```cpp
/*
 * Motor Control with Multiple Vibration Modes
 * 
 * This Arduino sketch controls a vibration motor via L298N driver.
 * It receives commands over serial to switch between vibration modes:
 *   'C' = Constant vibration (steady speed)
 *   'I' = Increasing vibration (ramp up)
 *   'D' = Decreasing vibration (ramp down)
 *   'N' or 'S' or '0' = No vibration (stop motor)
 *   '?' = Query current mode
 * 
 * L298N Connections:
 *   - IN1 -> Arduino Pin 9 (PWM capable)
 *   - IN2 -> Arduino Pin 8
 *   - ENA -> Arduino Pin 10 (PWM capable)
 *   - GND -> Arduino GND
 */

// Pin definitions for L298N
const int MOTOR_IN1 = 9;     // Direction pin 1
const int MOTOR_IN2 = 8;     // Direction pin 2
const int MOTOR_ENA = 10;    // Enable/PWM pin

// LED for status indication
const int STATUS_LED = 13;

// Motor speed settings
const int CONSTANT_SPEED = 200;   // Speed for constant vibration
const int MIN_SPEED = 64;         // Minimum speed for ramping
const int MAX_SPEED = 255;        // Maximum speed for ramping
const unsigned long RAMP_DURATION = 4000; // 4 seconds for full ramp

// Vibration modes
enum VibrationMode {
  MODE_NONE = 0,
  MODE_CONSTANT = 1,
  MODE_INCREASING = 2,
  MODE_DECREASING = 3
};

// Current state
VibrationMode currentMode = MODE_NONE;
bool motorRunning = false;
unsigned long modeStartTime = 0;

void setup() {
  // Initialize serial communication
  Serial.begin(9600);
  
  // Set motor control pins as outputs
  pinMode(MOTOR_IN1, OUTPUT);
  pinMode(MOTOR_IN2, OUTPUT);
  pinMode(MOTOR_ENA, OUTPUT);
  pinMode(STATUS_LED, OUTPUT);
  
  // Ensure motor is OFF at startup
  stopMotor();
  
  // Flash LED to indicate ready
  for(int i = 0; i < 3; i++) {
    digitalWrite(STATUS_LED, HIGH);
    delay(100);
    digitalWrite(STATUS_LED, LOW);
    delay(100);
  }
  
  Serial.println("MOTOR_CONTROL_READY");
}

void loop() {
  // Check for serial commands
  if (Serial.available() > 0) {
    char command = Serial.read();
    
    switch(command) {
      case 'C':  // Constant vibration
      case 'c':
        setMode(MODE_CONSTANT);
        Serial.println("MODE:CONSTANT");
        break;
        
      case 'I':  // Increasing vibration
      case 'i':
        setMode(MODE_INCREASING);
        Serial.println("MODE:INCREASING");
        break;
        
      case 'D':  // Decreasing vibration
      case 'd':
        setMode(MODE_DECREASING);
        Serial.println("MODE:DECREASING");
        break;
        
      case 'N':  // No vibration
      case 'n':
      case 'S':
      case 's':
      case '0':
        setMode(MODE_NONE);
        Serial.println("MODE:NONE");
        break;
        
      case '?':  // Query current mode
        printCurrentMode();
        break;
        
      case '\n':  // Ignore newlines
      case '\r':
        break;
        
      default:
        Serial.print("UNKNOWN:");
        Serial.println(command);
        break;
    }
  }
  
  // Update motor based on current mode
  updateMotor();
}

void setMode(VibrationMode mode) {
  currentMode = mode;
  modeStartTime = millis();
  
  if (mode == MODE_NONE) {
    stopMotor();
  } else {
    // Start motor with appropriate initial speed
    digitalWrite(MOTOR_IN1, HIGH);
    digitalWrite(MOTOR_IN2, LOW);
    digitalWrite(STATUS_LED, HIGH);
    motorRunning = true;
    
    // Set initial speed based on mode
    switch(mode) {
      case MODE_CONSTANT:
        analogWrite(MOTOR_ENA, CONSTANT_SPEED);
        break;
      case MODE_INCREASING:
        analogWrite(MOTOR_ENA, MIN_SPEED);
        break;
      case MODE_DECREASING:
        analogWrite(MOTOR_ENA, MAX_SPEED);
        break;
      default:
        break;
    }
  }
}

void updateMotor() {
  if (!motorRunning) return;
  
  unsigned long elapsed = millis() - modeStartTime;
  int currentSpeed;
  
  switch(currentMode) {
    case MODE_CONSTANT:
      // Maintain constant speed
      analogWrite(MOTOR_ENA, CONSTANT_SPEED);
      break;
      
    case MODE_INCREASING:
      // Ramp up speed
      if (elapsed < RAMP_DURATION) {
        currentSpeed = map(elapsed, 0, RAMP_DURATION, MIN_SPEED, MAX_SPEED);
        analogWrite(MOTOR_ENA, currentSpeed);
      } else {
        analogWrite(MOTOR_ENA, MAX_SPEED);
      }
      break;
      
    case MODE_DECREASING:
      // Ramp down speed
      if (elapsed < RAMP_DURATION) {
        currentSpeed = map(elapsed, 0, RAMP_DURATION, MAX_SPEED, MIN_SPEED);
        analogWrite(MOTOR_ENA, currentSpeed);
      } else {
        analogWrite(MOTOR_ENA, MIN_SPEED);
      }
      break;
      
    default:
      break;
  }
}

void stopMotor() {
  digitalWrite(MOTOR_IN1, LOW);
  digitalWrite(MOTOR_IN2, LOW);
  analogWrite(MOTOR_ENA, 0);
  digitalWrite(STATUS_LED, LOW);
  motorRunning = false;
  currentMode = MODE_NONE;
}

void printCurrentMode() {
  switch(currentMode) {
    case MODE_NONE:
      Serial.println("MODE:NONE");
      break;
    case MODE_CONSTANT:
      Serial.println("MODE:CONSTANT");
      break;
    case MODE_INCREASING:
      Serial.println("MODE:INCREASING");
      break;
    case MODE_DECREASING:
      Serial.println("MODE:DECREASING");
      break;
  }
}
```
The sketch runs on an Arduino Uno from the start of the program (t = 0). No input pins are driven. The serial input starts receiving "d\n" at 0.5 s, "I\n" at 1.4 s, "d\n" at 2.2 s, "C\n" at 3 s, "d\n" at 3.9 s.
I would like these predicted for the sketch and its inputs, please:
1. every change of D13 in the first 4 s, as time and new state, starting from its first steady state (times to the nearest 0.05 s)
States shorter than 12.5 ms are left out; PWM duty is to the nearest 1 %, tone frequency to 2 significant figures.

0 s high; 0.1 s low; 0.2 s high; 0.3 s low; 0.4 s high; 0.5 s low; 0.6 s high
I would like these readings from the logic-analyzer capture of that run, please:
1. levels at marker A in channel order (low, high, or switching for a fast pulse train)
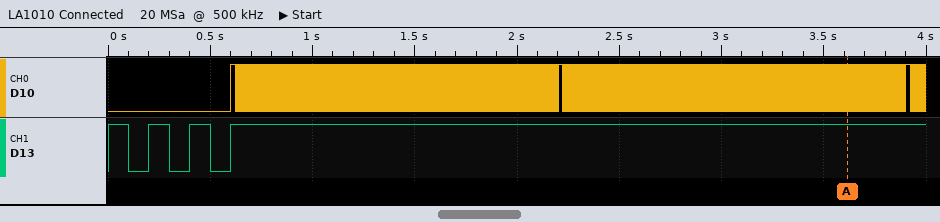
D10 switching, D13 high
